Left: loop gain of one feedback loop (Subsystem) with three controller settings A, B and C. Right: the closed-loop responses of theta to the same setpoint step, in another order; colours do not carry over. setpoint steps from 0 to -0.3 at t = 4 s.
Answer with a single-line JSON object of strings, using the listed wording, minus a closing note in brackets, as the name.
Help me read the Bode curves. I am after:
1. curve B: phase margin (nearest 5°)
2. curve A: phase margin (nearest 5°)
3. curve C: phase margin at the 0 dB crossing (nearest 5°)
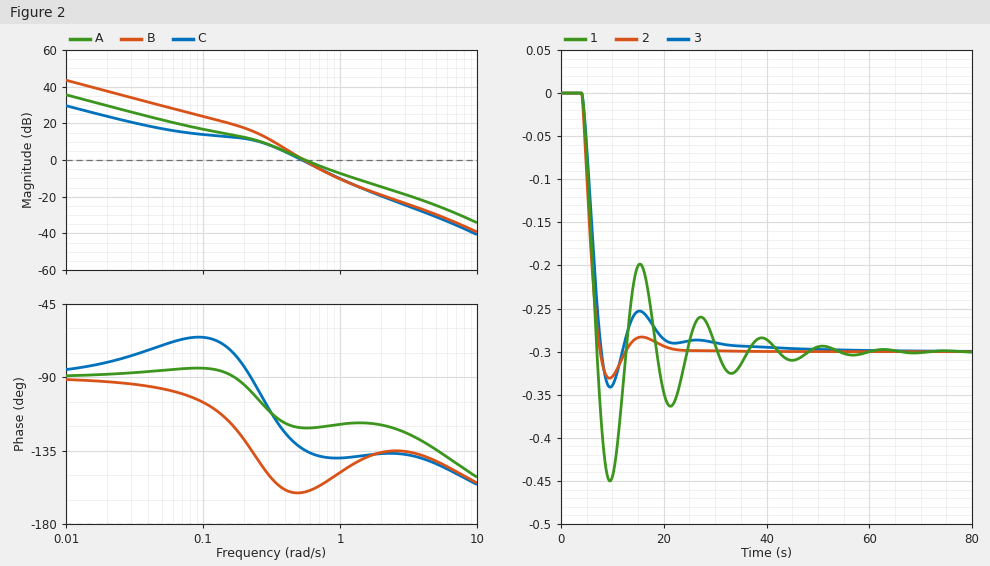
{"curve B: phase margin": "20°", "curve A: phase margin": "60°", "curve C: phase margin at the 0 dB crossing": "45°"}
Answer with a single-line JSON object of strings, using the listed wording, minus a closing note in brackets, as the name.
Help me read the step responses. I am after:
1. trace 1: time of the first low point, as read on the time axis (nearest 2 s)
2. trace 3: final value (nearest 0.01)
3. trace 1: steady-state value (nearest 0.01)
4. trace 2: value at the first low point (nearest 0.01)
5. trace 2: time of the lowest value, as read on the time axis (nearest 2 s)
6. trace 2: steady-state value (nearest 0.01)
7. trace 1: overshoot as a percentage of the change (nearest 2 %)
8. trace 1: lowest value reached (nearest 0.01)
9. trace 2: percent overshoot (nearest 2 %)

{"trace 1: time of the first low point, as read on the time axis": "10 s", "trace 3: final value": "-0.30", "trace 1: steady-state value": "-0.30", "trace 2: value at the first low point": "-0.33", "trace 2: time of the lowest value, as read on the time axis": "10 s", "trace 2: steady-state value": "-0.30", "trace 1: overshoot as a percentage of the change": "50 %", "trace 1: lowest value reached": "-0.45", "trace 2: percent overshoot": "10 %"}
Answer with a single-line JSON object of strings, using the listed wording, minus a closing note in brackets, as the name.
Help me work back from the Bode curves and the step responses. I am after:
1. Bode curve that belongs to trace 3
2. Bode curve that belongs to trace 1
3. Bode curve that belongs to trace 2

{"Bode curve that belongs to trace 3": "C", "Bode curve that belongs to trace 1": "B", "Bode curve that belongs to trace 2": "A"}
